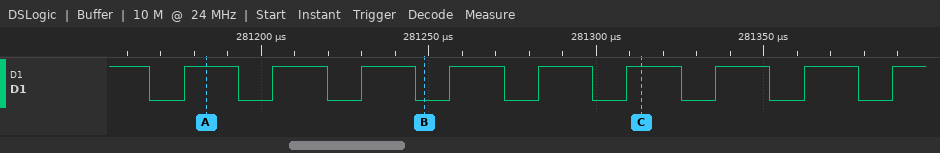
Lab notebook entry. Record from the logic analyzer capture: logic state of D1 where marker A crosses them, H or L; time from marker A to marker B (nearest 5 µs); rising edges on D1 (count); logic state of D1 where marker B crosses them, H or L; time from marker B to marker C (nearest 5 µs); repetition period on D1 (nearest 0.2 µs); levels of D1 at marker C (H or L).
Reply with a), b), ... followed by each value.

a) D1=H
b) 65 µs
c) 9
d) D1=L
e) 65 µs
f) 26.4 µs
g) D1=H
